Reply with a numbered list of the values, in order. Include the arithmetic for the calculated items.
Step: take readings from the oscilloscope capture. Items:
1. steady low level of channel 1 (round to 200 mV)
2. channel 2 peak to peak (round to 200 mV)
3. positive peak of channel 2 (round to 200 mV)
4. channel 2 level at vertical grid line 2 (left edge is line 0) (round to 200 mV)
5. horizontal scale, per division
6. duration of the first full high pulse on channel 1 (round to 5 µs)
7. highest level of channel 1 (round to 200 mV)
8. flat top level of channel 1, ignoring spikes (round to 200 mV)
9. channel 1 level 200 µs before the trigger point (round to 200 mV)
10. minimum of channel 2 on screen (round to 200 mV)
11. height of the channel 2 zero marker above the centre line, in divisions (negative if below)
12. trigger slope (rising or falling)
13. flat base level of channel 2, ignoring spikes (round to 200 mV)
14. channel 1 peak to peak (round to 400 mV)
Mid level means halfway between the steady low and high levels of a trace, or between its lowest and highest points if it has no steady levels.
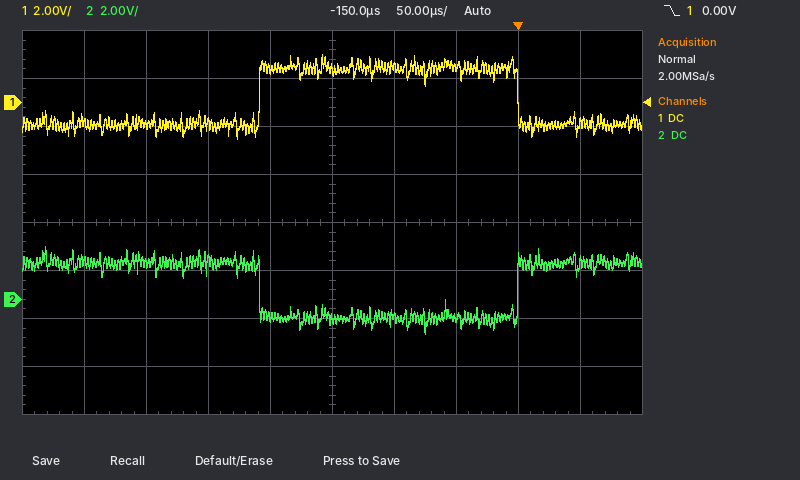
1. -1.0 V
2. 2.2 V − (-1.4 V) = 3.6 V
3. 2.2 V
4. 1.6 V
5. 50 µs
6. 210 µs
7. 2.0 V
8. 1.4 V
9. 1.4 V
10. -1.4 V
11. -1.6 div
12. falling
13. -800 mV
14. 3.6 V
